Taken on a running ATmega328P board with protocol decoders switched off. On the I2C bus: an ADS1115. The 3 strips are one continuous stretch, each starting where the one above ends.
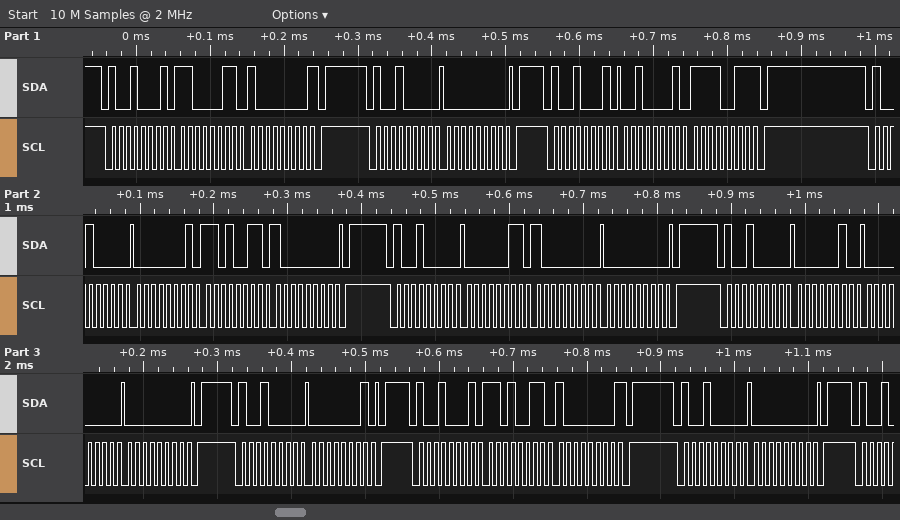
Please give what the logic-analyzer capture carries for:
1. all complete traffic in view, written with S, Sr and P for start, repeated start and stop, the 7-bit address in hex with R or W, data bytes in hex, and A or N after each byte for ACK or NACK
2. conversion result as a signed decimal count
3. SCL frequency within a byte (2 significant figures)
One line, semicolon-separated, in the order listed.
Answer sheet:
S 48R A C3 A 80 N P S 48W A 00 A P S 48R A 21 A F3 N P S 48W A 01 A D3 A 80 A P S 48W A 03 A 80 A 00 A P S 48W A 02 A 00 A 00 A P S 48W A 01 A P S 48R A D3 A 80 N P S 48W A 00 A P; 8691; 100 kHz
